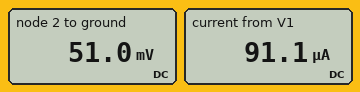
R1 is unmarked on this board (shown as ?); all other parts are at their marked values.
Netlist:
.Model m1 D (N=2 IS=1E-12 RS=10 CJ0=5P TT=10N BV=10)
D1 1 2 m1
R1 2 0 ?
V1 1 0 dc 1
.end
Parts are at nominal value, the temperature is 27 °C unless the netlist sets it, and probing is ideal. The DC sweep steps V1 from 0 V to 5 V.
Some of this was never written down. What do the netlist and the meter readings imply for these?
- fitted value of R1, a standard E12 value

560 Ω
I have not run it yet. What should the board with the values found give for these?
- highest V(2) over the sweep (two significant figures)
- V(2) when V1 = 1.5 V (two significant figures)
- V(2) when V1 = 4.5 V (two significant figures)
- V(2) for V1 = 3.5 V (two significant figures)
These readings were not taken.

3.8 V
430 mV
3.3 V
2.3 V
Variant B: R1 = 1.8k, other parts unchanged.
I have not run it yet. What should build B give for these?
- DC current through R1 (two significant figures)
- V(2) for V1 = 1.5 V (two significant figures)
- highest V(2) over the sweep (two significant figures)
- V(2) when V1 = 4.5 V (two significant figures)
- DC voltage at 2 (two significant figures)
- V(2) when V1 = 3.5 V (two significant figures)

47 µA
490 mV
3.9 V
3.4 V
85 mV
2.4 V
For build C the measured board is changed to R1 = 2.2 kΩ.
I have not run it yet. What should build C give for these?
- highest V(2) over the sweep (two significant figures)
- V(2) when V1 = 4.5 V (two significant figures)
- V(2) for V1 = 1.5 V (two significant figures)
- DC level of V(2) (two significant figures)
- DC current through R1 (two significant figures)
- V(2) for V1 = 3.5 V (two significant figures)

3.9 V
3.4 V
500 mV
92 mV
42 µA
2.4 V
